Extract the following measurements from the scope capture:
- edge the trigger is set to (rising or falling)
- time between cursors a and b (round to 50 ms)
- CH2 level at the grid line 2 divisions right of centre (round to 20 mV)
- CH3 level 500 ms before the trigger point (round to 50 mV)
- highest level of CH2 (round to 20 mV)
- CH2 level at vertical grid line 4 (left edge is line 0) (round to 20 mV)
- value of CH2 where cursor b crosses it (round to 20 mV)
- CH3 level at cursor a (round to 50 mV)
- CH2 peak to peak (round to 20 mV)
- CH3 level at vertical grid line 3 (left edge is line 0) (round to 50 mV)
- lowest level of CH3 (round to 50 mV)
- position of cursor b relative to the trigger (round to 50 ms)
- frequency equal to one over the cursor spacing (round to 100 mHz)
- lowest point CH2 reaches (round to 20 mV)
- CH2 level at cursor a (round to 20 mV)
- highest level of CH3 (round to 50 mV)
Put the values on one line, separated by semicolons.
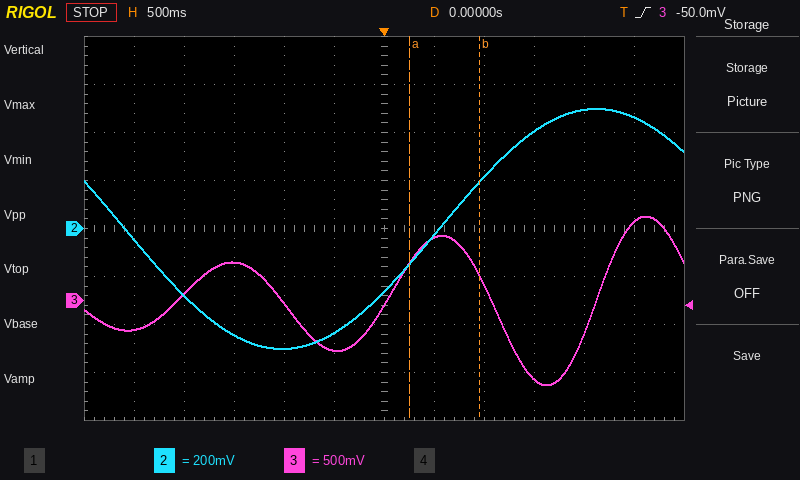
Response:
rising; 700 ms; 220 mV; -500 mV; 500 mV; -500 mV; 200 mV; 400 mV; 1.00 V; 400 mV; -900 mV; +950 ms; 1.4 Hz; -500 mV; -140 mV; 900 mV
